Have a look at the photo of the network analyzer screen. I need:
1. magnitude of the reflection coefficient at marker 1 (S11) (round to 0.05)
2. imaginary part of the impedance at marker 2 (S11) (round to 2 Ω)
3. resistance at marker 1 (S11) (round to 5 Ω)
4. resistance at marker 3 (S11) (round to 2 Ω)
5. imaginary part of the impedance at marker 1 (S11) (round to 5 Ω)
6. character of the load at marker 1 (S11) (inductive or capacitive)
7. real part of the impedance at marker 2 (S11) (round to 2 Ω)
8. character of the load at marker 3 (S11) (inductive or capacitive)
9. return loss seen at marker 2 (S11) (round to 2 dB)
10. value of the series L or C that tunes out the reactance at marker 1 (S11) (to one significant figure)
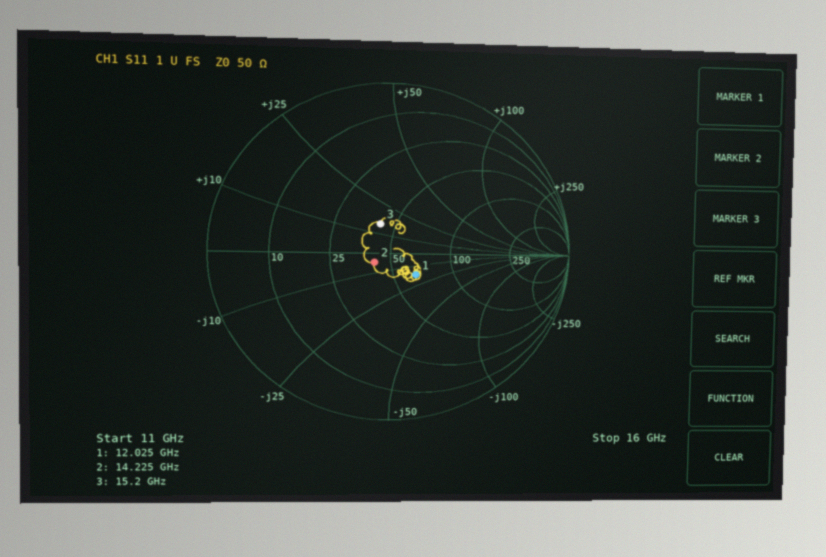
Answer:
0.20
-4 Ω
65 Ω
42 Ω
-15 Ω
capacitive
42 Ω
inductive
20 dB
200 pH
